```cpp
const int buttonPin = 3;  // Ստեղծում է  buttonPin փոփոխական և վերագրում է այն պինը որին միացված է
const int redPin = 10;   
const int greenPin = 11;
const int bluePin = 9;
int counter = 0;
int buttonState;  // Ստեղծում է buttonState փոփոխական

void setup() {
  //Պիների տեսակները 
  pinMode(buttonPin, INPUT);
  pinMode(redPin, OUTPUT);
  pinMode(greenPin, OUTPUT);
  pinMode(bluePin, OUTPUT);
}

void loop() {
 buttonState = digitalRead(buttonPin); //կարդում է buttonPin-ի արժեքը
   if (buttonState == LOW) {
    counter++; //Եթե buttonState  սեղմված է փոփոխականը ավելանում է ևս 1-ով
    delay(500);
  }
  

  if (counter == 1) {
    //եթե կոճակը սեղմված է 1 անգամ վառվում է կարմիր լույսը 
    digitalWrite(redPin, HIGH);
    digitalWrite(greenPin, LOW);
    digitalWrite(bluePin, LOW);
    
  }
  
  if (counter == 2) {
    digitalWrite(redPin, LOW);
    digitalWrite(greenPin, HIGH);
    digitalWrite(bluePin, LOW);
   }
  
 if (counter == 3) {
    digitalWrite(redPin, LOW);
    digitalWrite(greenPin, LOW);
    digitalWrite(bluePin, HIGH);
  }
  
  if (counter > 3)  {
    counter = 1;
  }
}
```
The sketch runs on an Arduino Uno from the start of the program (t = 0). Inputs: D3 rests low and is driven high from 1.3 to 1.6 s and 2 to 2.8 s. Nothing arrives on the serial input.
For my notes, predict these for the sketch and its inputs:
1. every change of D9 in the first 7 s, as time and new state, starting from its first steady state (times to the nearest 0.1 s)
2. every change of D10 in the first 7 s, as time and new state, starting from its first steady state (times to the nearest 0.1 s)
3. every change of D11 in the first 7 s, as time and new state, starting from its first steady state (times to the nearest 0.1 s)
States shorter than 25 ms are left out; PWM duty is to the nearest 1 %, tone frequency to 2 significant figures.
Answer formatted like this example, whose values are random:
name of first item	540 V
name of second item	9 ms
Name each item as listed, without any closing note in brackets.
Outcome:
every change of D9 in the first 7 s, as time and new state, starting from its first steady state	0 s low; 1.5 s high; 2.1 s low; 3.8 s high; 4.8 s low; 5.3 s high; 6.3 s low; 6.8 s high
every change of D10 in the first 7 s, as time and new state, starting from its first steady state	0 s low; 0.5 s high; 1 s low; 2.1 s high; 3.3 s low
every change of D11 in the first 7 s, as time and new state, starting from its first steady state	0 s low; 1 s high; 1.5 s low; 3.3 s high; 3.8 s low; 4.8 s high; 5.3 s low; 6.3 s high; 6.8 s low
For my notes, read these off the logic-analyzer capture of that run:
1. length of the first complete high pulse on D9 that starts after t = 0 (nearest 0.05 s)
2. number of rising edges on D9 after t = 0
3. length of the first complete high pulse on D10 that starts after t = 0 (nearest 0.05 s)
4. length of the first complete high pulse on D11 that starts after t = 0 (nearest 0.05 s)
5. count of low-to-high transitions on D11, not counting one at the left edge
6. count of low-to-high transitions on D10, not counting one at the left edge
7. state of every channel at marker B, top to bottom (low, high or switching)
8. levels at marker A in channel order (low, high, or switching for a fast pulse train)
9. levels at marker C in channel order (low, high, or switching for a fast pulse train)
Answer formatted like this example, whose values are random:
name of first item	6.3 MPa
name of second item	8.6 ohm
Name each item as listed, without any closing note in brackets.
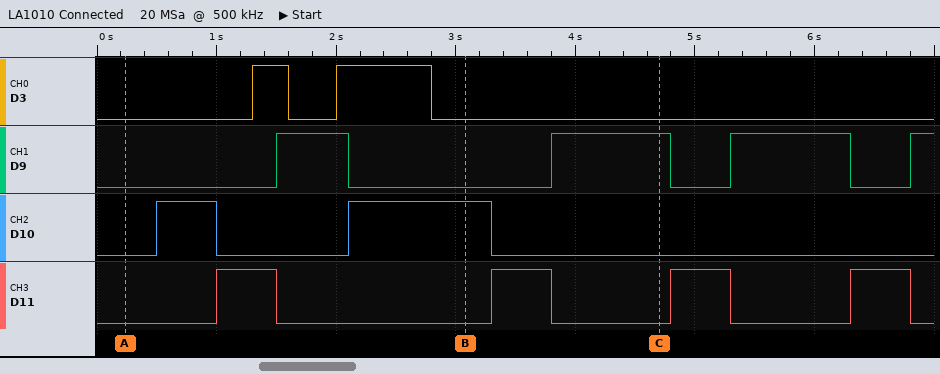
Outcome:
length of the first complete high pulse on D9 that starts after t = 0	0.60 s
number of rising edges on D9 after t = 0	4
length of the first complete high pulse on D10 that starts after t = 0	0.50 s
length of the first complete high pulse on D11 that starts after t = 0	0.50 s
count of low-to-high transitions on D11, not counting one at the left edge	4
count of low-to-high transitions on D10, not counting one at the left edge	2
state of every channel at marker B, top to bottom	D3 low, D9 low, D10 high, D11 low
levels at marker A in channel order	D3 low, D9 low, D10 low, D11 low
levels at marker C in channel order	D3 low, D9 high, D10 low, D11 low
